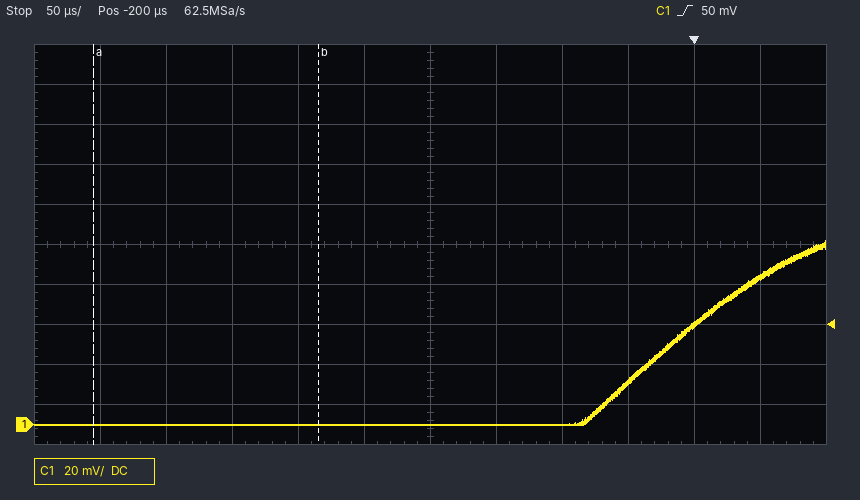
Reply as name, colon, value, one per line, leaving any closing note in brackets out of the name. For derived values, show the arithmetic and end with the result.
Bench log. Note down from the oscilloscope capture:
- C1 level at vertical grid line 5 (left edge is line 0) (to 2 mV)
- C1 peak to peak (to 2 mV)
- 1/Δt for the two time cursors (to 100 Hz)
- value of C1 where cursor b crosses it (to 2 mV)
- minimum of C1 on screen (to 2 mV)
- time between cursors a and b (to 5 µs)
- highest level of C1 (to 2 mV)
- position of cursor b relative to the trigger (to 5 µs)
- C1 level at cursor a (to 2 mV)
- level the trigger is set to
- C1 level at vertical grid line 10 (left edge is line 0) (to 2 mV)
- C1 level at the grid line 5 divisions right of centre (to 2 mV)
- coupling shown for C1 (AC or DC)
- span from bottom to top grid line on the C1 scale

C1 level at vertical grid line 5 (left edge is line 0): 0 mV
C1 peak to peak: 92 mV − (0 mV) = 92 mV
1/Δt for the two time cursors: 1 / 170 µs ≈ 5.9 kHz
value of C1 where cursor b crosses it: 0 mV
minimum of C1 on screen: 0 mV
time between cursors a and b: 170 µs
highest level of C1: 92 mV
position of cursor b relative to the trigger: -285 µs
C1 level at cursor a: 0 mV
level the trigger is set to: 50 mV
C1 level at vertical grid line 10 (left edge is line 0): 50 mV
C1 level at the grid line 5 divisions right of centre: 74 mV
coupling shown for C1: DC
span from bottom to top grid line on the C1 scale: 200 mV
